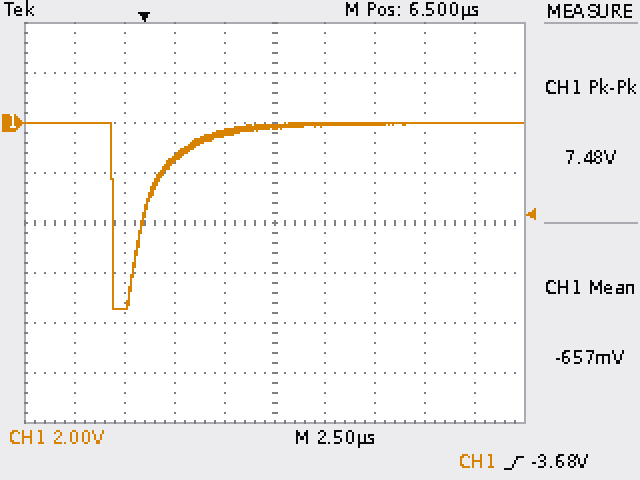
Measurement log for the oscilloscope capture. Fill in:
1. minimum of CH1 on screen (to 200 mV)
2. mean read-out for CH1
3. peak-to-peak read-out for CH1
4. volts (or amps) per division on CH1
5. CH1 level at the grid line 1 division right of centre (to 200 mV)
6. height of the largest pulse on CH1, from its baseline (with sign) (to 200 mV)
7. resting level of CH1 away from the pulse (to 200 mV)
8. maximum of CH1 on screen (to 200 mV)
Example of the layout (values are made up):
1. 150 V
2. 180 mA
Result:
1. -7.4 V
2. -657 mV
3. 7.48 V
4. 2 V
5. 0.0 V
6. -7.4 V
7. 0.0 V
8. 0.0 V
